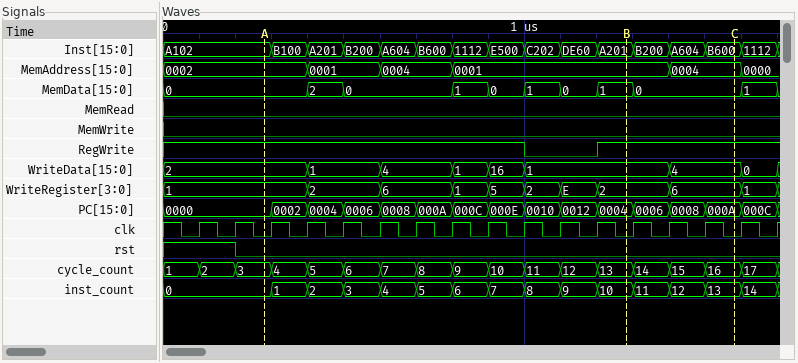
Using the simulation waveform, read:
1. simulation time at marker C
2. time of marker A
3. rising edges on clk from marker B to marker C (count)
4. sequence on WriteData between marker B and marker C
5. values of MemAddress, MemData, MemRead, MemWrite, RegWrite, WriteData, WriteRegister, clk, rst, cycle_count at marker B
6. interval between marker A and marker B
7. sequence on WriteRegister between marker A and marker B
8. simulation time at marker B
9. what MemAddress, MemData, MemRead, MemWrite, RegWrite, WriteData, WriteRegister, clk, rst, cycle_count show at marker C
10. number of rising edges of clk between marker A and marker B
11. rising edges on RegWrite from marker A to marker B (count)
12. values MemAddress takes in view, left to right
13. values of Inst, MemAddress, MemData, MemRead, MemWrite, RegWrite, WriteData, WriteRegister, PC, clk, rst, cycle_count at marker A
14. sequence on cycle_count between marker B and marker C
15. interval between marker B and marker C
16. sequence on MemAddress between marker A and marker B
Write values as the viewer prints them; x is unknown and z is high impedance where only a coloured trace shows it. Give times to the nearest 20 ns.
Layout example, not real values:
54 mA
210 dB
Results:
1580 ns
280 ns
3
1, 4
MemAddress=0001, MemData=1, MemRead=0, MemWrite=0, RegWrite=1, WriteData=1, WriteRegister=2, clk=0, rst=0, cycle_count=13
1000 ns
1, 2, 6, 1, 5, 2, E, 2
1280 ns
MemAddress=0004, MemData=0, MemRead=0, MemWrite=0, RegWrite=1, WriteData=4, WriteRegister=6, clk=0, rst=0, cycle_count=16
10
1
0002, 0001, 0004, 0001, 0004, 0000
Inst=A102, MemAddress=0002, MemData=0, MemRead=0, MemWrite=0, RegWrite=1, WriteData=2, WriteRegister=1, PC=0000, clk=0, rst=0, cycle_count=3
13, 14, 15, 16
300 ns
0002, 0001, 0004, 0001
